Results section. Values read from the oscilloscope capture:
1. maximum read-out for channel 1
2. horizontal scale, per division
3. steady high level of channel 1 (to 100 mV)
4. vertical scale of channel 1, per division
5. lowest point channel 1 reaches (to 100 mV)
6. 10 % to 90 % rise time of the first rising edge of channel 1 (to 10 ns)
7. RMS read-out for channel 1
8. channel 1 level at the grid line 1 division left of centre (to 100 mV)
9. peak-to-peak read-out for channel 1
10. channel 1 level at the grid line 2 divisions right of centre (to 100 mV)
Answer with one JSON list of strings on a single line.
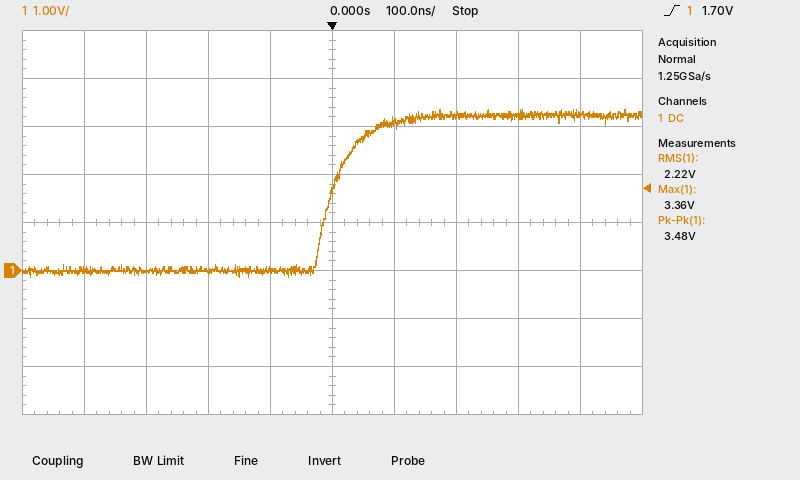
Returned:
["3.36 V", "100 ns", "3.2 V", "1 V", "-100 mV", "90 ns", "2.22 V", "0.0 V", "3.48 V", "3.2 V"]
